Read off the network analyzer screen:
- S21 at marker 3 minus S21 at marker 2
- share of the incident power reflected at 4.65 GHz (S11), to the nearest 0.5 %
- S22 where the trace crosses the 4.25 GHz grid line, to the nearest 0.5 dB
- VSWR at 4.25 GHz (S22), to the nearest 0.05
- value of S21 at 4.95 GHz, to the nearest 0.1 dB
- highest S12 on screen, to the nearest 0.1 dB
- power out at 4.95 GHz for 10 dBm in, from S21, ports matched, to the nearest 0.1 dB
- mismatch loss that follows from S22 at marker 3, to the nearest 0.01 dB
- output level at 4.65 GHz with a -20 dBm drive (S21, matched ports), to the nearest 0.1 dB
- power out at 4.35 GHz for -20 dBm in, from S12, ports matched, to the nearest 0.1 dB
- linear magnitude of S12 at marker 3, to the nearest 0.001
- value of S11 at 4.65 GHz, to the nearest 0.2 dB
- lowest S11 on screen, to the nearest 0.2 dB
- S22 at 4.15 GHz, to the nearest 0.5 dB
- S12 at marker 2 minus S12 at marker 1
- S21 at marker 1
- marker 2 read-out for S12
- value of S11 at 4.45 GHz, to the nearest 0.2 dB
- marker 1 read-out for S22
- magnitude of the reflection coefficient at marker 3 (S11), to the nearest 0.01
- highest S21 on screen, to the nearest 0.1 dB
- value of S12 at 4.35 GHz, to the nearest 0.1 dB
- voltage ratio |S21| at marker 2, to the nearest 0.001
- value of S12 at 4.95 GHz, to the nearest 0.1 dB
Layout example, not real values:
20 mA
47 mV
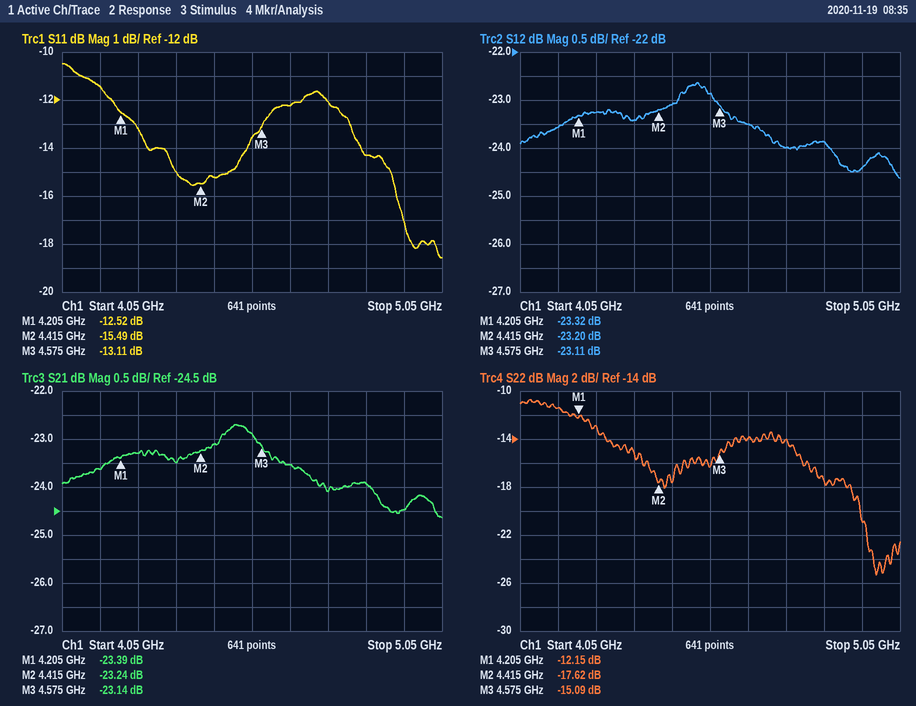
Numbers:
0.10 dB
6.0 %
-13.0 dB
1.60
-24.5 dB
-22.6 dB
-14.5 dBm
0.14 dB
-43.5 dBm
-43.4 dBm
0.070
-12.2 dB
-18.6 dB
-11.5 dB
0.12 dB
-23.39 dB
-23.20 dB
-15.2 dB
-12.15 dB
0.22
-22.7 dB
-23.4 dB
0.069
-24.4 dB
